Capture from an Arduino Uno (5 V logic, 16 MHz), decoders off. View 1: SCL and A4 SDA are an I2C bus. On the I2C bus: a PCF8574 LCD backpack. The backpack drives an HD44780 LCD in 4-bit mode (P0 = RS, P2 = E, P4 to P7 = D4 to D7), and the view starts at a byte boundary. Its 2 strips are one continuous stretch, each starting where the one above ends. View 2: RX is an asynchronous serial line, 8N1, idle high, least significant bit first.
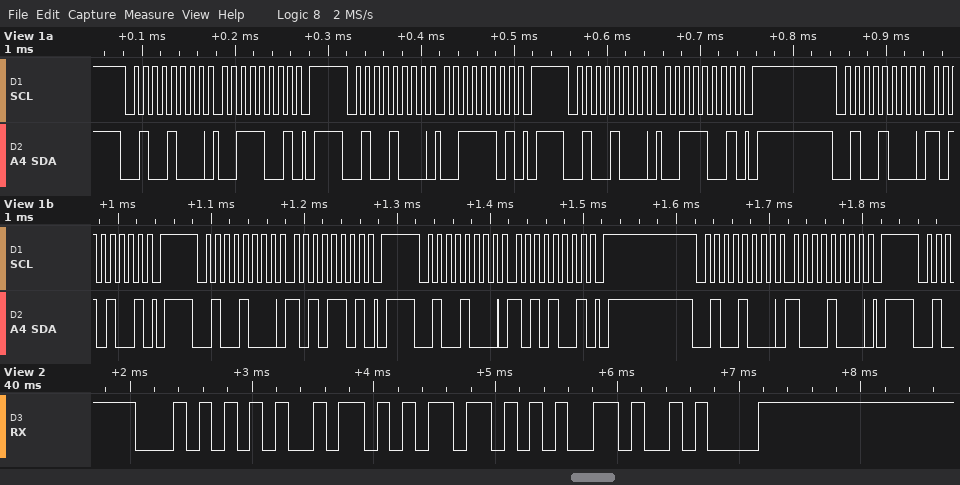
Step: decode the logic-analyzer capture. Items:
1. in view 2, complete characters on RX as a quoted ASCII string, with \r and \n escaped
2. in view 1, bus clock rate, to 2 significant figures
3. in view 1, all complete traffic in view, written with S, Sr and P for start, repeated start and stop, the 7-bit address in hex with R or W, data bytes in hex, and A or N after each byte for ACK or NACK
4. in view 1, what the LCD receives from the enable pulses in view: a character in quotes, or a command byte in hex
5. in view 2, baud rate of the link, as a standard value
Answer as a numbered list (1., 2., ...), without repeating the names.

1. "Time\n"
2. 100 kHz
3. S 24W A 39 A P S 24W A 3D A P S 24W A 39 A P S 24W A A9 A P S 24W A AD A P S 24W A A9 A P S 24W A 88 A P
4. ':'
5. 9600 baud
